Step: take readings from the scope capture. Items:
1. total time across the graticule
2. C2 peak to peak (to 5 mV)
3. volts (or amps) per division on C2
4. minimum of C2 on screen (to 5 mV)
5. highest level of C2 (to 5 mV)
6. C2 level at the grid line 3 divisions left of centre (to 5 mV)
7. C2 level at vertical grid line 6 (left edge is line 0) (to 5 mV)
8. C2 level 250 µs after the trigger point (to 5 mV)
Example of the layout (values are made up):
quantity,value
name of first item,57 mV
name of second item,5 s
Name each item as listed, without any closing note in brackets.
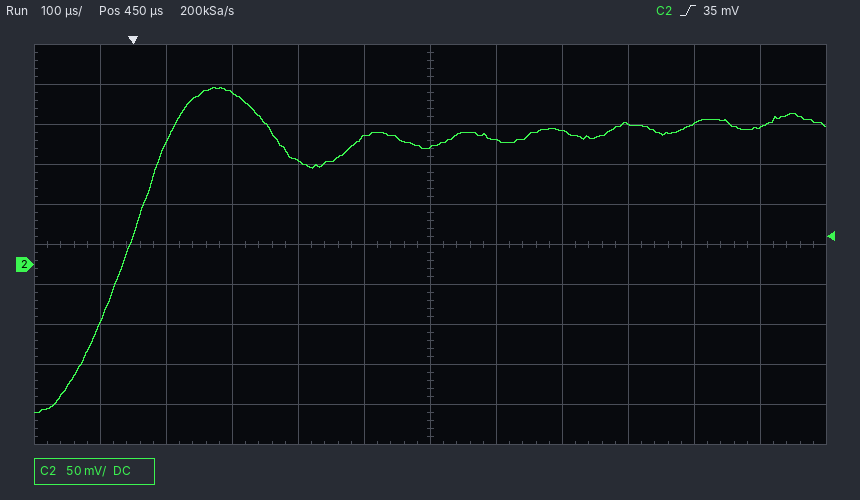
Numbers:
quantity,value
total time across the graticule,1.2 ms
C2 peak to peak,405 mV
volts (or amps) per division on C2,50 mV
minimum of C2 on screen,-185 mV
highest level of C2,220 mV
C2 level at the grid line 3 divisions left of centre,215 mV
C2 level at vertical grid line 6 (left edge is line 0),145 mV
C2 level 250 µs after the trigger point,130 mV
